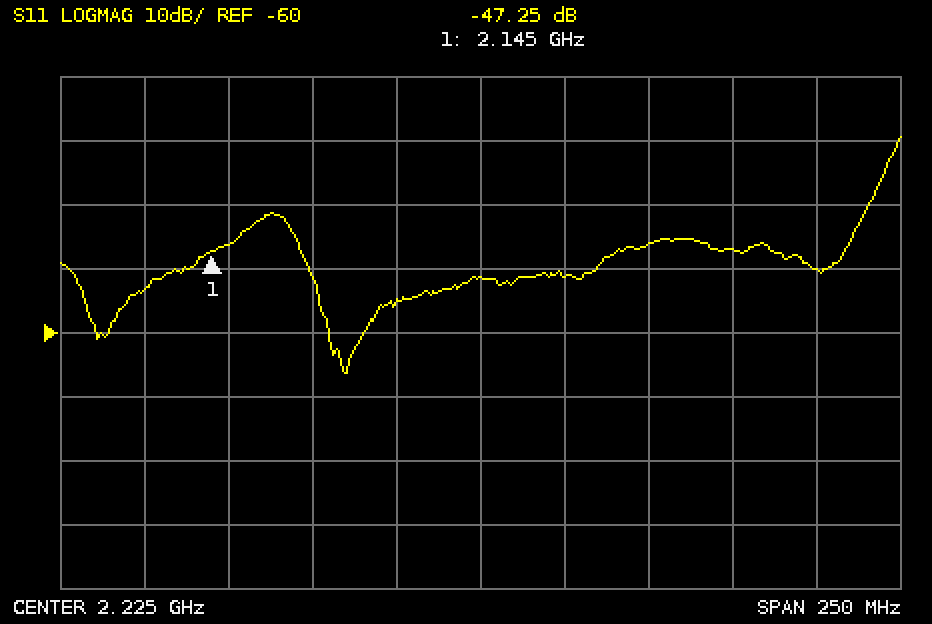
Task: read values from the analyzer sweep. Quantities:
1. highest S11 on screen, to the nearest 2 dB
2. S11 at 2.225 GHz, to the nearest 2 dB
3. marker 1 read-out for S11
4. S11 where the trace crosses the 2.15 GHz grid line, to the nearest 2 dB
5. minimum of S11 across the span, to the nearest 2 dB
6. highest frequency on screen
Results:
-30 dB
-52 dB
-47.25 dB
-46 dB
-66 dB
2.35 GHz
